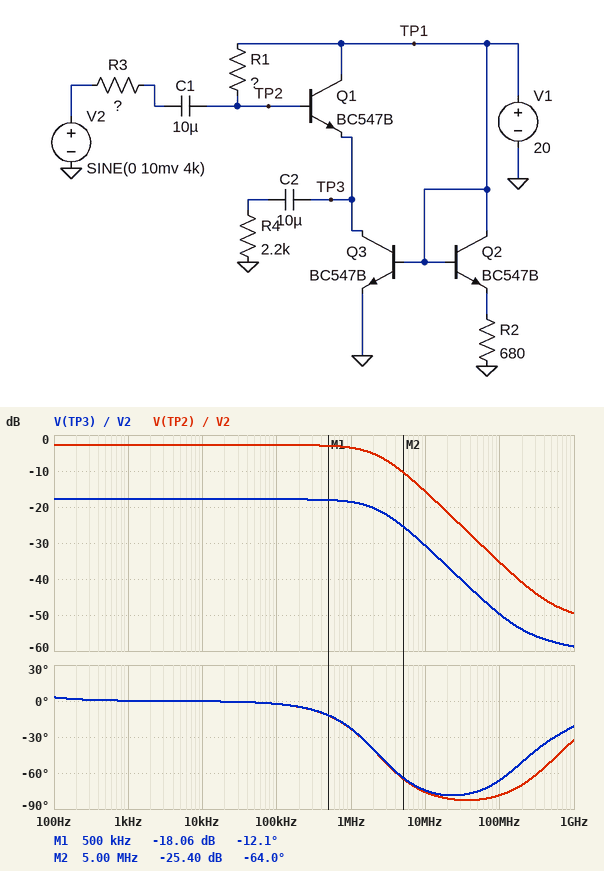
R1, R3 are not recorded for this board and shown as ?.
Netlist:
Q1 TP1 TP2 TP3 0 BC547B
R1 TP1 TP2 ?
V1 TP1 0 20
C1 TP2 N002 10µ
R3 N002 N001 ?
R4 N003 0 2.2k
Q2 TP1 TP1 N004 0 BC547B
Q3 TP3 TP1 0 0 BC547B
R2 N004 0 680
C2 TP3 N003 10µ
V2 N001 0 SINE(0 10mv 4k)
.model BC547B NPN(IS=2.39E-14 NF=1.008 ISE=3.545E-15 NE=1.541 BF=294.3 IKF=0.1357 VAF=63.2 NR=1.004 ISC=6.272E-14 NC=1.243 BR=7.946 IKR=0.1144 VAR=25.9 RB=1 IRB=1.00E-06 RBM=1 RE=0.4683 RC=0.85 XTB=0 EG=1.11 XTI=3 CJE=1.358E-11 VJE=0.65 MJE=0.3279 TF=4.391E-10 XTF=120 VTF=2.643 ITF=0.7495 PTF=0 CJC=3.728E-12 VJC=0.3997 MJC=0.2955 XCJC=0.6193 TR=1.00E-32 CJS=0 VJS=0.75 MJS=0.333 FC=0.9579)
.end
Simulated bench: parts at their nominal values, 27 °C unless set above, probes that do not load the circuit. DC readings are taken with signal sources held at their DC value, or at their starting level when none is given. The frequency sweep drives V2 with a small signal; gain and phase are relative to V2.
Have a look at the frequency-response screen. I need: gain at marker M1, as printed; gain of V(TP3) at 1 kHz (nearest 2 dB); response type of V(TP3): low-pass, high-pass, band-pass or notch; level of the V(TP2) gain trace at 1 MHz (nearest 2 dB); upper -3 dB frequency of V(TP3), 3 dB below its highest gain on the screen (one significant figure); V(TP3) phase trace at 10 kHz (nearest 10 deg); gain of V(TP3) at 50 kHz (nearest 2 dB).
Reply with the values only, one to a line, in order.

-18.06 dB
-18 dB
low-pass
-4 dB
2 MHz
0 deg
-18 dB
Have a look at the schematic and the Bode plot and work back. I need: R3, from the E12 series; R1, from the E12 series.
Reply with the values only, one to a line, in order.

820 Ω
820 kΩ
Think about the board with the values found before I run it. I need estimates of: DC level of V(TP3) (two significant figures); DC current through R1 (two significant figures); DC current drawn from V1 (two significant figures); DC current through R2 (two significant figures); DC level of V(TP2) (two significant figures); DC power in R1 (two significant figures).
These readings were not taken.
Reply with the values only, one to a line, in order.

6.1 V
16 µA
13 A
28 mA
6.8 V
210 µW
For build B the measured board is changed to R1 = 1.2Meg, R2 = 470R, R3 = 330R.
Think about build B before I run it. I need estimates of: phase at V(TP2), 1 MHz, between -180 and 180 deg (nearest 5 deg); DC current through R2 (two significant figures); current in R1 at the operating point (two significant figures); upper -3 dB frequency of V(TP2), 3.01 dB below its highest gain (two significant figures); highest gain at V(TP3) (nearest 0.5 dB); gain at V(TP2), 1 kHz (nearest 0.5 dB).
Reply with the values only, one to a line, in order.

-10 deg
41 mA
11 µA
5.4 MHz
-18.5 dB
-1.0 dB
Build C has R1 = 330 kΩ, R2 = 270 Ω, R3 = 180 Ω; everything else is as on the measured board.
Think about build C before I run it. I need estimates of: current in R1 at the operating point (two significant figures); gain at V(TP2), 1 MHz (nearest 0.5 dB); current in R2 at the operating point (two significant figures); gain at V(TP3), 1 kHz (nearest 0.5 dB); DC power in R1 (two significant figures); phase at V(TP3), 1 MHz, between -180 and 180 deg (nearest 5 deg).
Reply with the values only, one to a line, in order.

40 µA
-1.5 dB
71 mA
-11.5 dB
520 µW
-10 deg
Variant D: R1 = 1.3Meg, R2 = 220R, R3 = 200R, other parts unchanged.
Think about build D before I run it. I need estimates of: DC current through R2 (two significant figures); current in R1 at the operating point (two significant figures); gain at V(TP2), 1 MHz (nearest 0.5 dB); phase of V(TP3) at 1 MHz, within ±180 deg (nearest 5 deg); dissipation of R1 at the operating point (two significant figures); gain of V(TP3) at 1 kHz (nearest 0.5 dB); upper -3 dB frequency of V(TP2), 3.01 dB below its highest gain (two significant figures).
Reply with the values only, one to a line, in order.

87 mA
10 µA
-0.5 dB
-5 deg
130 µW
-18.5 dB
8.7 MHz
